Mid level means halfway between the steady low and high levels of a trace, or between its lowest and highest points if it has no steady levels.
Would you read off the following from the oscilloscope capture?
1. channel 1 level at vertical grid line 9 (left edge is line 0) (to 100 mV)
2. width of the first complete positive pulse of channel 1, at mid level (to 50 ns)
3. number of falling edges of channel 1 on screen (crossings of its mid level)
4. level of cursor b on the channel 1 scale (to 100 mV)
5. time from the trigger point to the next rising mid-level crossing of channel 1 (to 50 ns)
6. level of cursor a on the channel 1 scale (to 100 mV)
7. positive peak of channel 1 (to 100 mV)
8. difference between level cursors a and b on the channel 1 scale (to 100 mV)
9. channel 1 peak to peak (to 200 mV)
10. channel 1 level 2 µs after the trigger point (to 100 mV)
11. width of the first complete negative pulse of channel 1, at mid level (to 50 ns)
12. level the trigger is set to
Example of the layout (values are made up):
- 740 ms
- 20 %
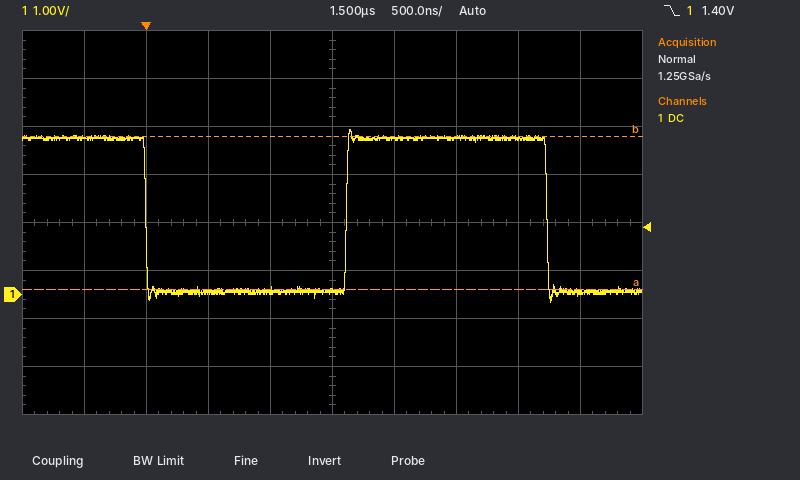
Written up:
- 0.0 V
- 1.60 µs
- 2
- 3.3 V
- 1.60 µs
- 100 mV
- 3.4 V
- 3.2 V
- 3.6 V
- 3.2 V
- 1.60 µs
- 1.40 V
